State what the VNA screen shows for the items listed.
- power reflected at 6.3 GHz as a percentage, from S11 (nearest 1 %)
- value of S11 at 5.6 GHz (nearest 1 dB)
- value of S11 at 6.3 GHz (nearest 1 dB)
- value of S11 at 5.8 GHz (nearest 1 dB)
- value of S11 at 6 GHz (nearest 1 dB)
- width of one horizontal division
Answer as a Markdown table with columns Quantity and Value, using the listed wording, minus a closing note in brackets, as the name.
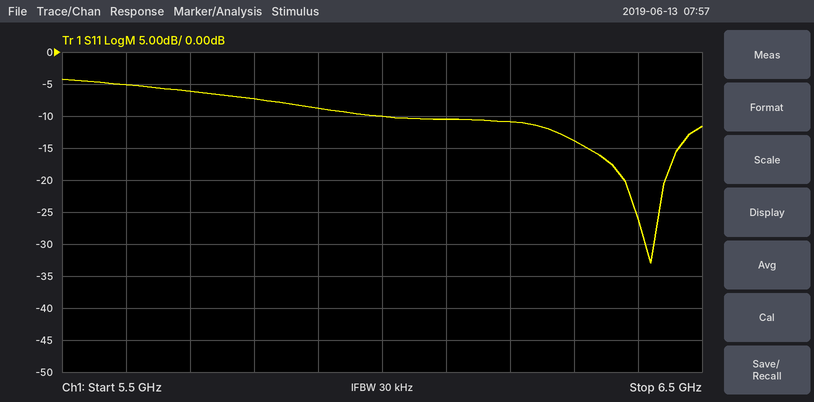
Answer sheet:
| Quantity | Value |
|---|---|
| power reflected at 6.3 GHz as a percentage, from S11 | 4 % |
| value of S11 at 5.6 GHz | -5 dB |
| value of S11 at 6.3 GHz | -14 dB |
| value of S11 at 5.8 GHz | -7 dB |
| value of S11 at 6 GHz | -10 dB |
| width of one horizontal division | 100 MHz |
